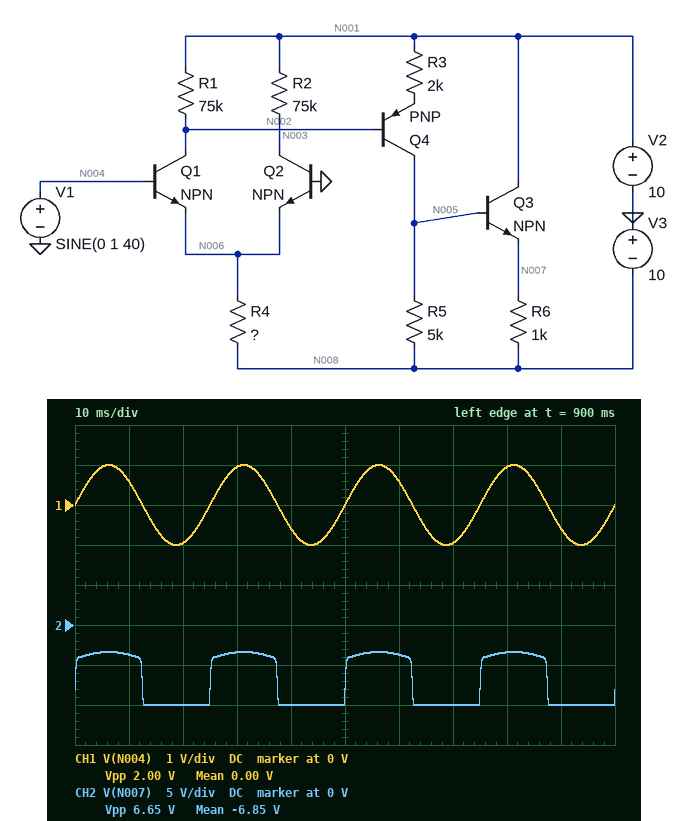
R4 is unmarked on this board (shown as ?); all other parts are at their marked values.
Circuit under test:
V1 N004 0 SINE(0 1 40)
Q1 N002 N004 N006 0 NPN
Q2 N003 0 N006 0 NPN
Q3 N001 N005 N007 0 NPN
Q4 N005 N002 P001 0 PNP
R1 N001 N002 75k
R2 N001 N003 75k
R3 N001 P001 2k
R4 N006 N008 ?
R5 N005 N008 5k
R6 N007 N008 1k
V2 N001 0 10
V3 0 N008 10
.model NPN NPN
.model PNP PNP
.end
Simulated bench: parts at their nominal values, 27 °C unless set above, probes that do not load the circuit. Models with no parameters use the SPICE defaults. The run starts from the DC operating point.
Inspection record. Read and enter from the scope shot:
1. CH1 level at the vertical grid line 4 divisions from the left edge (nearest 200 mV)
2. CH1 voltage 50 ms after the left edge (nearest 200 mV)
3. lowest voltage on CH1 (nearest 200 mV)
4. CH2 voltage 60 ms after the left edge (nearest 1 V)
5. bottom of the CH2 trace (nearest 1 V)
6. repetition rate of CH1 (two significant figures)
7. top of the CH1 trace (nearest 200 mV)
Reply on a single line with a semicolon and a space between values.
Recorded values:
-600 mV; 0 V; -1.0 V; -4 V; -10 V; 40 Hz; 1.0 V
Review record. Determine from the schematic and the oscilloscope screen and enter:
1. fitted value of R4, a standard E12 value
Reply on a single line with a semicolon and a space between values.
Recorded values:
150 kΩ
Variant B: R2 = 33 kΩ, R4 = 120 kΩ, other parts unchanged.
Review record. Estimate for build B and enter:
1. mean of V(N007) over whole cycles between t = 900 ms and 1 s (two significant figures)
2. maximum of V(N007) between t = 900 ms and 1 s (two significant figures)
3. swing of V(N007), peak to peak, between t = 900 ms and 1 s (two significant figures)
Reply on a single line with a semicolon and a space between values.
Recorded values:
-5.8 V; -1.2 V; 8.8 V
